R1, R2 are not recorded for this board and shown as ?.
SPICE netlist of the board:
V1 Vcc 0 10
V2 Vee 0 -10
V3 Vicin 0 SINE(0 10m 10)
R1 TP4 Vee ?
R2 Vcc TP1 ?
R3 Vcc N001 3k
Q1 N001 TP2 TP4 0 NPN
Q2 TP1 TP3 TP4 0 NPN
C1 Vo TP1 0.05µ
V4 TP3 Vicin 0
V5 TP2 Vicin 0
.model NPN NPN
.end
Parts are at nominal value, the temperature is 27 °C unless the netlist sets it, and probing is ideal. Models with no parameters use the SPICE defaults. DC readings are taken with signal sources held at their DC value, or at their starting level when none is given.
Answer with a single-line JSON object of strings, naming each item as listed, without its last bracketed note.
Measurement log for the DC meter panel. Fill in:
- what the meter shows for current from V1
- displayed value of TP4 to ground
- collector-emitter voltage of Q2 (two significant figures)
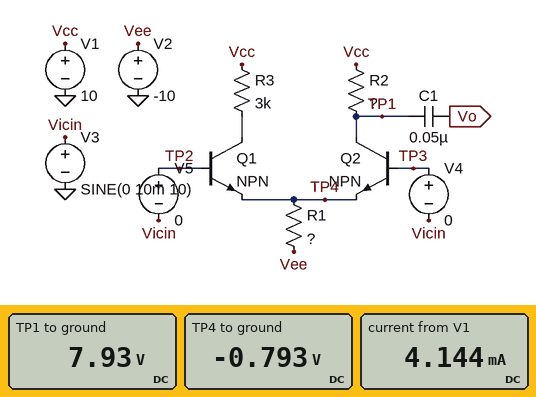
{"what the meter shows for current from V1": "4.144 mA", "displayed value of TP4 to ground": "-0.793 V", "collector-emitter voltage of Q2": "8.7 V"}
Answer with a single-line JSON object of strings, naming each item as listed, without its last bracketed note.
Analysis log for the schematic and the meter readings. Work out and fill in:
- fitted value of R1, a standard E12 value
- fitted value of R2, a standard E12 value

{"fitted value of R1, a standard E12 value": "2.2 kΩ", "fitted value of R2, a standard E12 value": "1 kΩ"}
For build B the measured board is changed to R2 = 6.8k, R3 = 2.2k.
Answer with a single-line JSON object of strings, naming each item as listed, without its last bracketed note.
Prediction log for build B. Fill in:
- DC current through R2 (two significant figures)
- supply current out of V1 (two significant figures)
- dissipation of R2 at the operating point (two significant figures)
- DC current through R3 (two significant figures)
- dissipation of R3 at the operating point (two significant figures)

{"DC current through R2": "1.6 mA", "supply current out of V1": "3.8 mA", "dissipation of R2 at the operating point": "17 mW", "DC current through R3": "2.2 mA", "dissipation of R3 at the operating point": "11 mW"}
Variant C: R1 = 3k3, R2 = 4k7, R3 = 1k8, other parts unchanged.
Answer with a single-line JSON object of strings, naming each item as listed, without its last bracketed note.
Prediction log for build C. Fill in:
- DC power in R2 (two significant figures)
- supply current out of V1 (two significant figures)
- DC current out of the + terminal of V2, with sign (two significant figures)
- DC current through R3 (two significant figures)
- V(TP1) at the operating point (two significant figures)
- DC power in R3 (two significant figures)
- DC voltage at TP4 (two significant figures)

{"DC power in R2": "9.0 mW", "supply current out of V1": "2.8 mA", "DC current out of the + terminal of V2, with sign": "-2.8 mA", "DC current through R3": "1.4 mA", "V(TP1) at the operating point": "3.5 V", "DC power in R3": "3.4 mW", "DC voltage at TP4": "-780 mV"}
